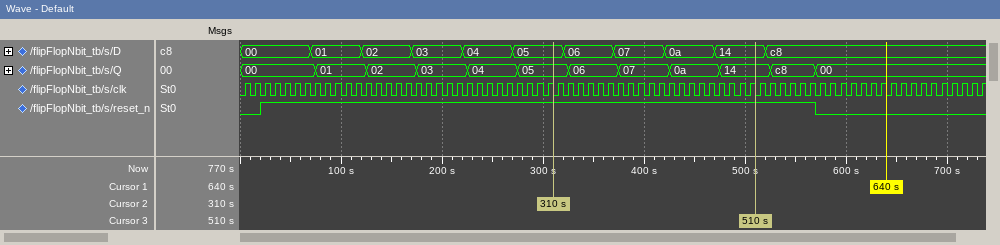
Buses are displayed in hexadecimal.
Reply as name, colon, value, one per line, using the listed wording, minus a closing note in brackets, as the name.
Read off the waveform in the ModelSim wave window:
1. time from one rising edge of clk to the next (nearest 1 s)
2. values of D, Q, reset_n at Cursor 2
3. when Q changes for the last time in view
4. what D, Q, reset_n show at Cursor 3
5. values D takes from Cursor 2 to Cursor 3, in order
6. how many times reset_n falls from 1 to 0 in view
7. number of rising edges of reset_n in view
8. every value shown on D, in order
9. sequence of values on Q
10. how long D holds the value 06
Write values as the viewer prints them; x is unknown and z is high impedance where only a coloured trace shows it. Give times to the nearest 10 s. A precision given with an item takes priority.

time from one rising edge of clk to the next: 10 s
values of D, Q, reset_n at Cursor 2: D=05, Q=05, reset_n=1
when Q changes for the last time in view: 570 s
what D, Q, reset_n show at Cursor 3: D=14, Q=14, reset_n=1
values D takes from Cursor 2 to Cursor 3, in order: 05, 06, 07, 0a, 14
how many times reset_n falls from 1 to 0 in view: 1
number of rising edges of reset_n in view: 1
every value shown on D, in order: 00, 01, 02, 03, 04, 05, 06, 07, 0a, 14, c8
sequence of values on Q: 00, 01, 02, 03, 04, 05, 06, 07, 0a, 14, c8, 00
how long D holds the value 06: 50 s
